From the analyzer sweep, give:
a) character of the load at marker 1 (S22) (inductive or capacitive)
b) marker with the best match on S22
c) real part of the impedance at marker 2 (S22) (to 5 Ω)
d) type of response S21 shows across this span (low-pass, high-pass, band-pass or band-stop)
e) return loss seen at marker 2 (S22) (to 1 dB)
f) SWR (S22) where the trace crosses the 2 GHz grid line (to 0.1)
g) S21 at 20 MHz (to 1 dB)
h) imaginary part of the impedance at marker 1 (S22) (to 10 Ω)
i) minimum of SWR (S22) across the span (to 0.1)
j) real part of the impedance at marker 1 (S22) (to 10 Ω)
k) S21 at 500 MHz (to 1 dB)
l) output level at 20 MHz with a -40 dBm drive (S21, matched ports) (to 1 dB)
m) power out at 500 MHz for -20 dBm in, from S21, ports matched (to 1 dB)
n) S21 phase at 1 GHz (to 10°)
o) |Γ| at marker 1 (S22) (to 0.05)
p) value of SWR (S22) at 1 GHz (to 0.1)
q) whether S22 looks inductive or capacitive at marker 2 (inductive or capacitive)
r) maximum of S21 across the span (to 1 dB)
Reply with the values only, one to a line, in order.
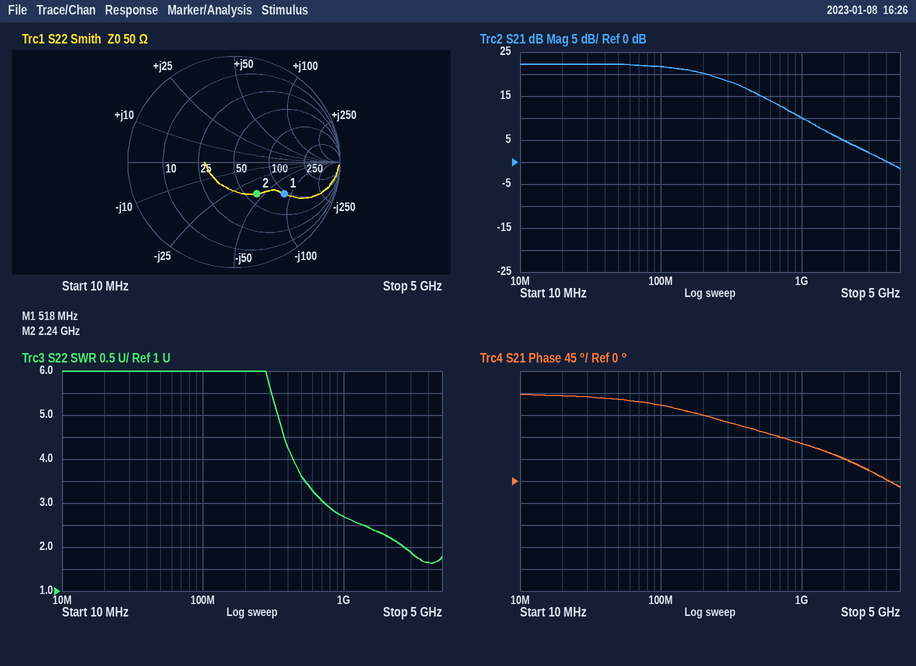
capacitive
marker 2
60 Ω
low-pass
9 dB
2.3
22 dB
-80 Ω
1.6
90 Ω
15 dB
-18 dBm
-5 dBm
80°
0.55
2.7
capacitive
22 dB
